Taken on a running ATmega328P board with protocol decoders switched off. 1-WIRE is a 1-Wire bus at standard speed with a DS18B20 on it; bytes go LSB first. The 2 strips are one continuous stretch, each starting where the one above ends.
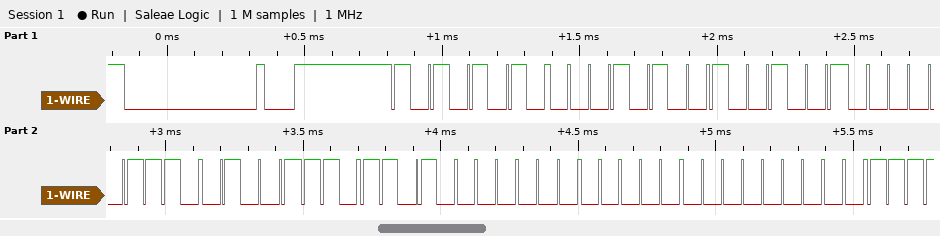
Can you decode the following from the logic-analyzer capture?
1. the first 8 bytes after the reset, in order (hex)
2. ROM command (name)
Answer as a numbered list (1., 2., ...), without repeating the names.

1. 55 28 49 70 72 0B 00 00
2. Match ROM
